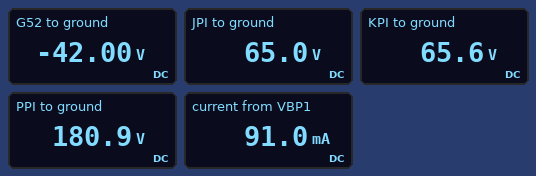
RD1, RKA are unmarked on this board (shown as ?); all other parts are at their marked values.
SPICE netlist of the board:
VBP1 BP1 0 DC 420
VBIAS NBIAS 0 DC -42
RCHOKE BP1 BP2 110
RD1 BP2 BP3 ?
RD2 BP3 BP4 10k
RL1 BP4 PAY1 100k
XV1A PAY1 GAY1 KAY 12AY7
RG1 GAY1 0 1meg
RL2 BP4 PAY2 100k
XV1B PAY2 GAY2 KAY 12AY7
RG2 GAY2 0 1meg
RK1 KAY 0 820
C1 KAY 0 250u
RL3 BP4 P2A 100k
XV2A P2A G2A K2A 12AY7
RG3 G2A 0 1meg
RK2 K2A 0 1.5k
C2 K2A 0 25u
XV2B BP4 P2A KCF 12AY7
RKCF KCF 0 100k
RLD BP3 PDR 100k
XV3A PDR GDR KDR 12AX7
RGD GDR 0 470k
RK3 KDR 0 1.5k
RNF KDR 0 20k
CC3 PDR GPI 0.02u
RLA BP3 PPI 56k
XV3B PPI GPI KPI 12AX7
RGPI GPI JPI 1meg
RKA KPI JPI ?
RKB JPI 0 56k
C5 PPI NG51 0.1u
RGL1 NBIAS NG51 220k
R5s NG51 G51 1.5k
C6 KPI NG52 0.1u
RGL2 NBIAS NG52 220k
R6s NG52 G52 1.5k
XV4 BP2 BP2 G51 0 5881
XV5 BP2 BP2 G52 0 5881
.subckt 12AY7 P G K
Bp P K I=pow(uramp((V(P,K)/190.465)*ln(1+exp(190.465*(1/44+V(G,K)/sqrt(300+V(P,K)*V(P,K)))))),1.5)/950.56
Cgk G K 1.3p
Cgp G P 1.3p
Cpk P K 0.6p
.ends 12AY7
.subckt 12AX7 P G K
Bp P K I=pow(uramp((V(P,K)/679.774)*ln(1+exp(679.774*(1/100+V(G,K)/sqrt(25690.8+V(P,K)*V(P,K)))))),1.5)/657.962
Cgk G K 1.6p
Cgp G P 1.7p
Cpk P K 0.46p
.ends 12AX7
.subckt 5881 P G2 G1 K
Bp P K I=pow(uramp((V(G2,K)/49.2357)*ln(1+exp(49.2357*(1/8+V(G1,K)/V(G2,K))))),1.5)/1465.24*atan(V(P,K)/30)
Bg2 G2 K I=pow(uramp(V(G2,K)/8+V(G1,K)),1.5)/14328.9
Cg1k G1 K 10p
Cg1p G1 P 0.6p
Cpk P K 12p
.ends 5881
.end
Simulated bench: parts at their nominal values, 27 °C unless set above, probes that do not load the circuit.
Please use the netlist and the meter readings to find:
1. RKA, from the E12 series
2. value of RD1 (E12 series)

470 Ω
27 kΩ
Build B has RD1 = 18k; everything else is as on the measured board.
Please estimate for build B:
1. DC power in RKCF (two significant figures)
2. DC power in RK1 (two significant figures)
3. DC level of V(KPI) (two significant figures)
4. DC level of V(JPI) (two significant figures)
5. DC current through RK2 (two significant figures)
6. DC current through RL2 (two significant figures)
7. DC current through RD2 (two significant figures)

150 mW
4.2 mW
76 V
75 V
1.2 mA
1.1 mA
4.7 mA
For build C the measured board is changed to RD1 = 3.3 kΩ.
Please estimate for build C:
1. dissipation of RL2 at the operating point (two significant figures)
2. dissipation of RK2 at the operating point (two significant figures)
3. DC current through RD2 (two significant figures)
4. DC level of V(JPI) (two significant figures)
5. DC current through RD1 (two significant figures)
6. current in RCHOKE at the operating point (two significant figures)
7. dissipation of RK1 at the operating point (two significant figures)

240 mW
3.8 mW
6.3 mA
100 V
9.4 mA
94 mA
7.8 mW
